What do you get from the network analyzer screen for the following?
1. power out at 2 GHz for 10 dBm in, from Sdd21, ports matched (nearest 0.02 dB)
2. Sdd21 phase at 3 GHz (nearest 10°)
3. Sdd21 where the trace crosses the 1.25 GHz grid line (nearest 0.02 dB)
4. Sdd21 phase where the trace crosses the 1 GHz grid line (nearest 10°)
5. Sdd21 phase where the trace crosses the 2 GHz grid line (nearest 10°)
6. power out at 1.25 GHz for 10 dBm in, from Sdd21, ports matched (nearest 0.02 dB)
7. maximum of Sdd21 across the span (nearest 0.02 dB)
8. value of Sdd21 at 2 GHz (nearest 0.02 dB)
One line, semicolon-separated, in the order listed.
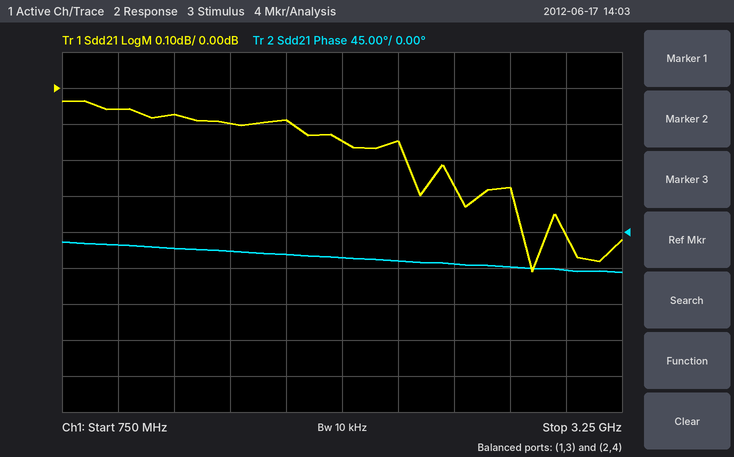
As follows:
9.86 dBm; -50°; -0.08 dB; -20°; -30°; 9.92 dBm; -0.04 dB; -0.14 dB
